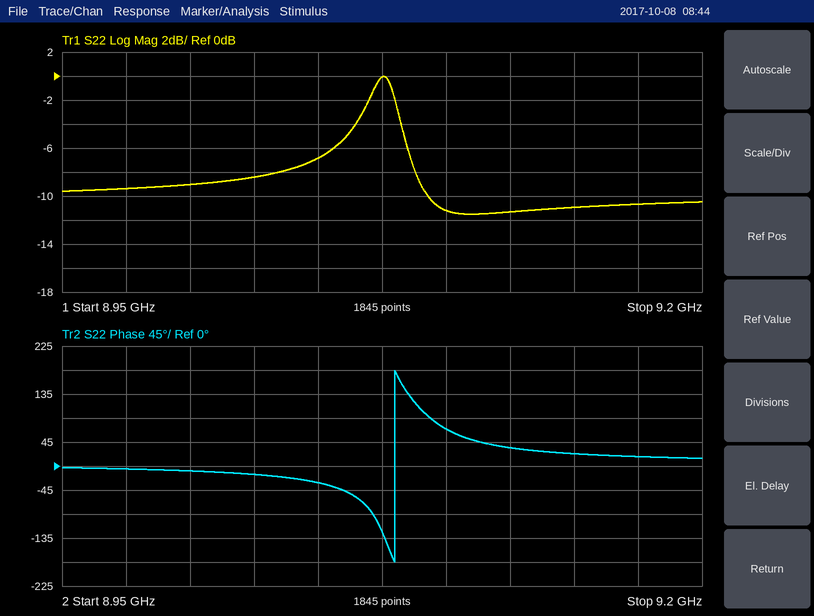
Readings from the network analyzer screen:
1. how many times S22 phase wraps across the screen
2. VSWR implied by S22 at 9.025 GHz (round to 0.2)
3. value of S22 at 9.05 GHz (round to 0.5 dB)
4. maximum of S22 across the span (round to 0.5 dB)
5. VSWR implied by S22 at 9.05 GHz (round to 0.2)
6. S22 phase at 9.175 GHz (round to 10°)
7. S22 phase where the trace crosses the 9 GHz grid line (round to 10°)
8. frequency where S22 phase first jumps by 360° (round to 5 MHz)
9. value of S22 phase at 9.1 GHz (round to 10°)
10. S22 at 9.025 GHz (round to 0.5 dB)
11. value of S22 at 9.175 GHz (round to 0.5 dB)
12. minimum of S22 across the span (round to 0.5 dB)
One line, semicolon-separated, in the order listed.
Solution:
1; 2.2; -7.0 dB; 0.0 dB; 2.6; 20°; -10°; 9.080 GHz; 70°; -8.5 dB; -10.5 dB; -11.5 dB
